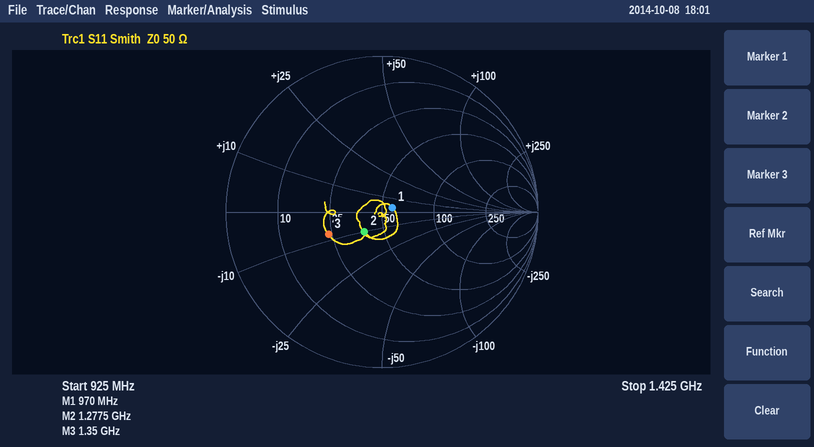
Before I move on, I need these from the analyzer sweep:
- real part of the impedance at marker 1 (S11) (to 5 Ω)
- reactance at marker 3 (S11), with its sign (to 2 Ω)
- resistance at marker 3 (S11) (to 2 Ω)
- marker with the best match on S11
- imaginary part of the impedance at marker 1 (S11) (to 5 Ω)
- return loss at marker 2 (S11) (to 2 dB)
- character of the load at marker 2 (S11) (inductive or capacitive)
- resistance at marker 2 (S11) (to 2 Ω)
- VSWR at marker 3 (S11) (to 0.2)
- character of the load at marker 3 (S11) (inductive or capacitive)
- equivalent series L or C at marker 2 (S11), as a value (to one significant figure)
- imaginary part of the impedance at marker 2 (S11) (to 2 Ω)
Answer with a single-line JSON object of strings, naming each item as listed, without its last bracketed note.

{"real part of the impedance at marker 1 (S11)": "55 Ω", "reactance at marker 3 (S11), with its sign": "-8 Ω", "resistance at marker 3 (S11)": "24 Ω", "marker with the best match on S11": "marker 1", "imaginary part of the impedance at marker 1 (S11)": "+5 Ω", "return loss at marker 2 (S11)": "16 dB", "character of the load at marker 2 (S11)": "capacitive", "resistance at marker 2 (S11)": "38 Ω", "VSWR at marker 3 (S11)": "2.2", "character of the load at marker 3 (S11)": "capacitive", "equivalent series L or C at marker 2 (S11), as a value": "10 pF", "imaginary part of the impedance at marker 2 (S11)": "-10 Ω"}
